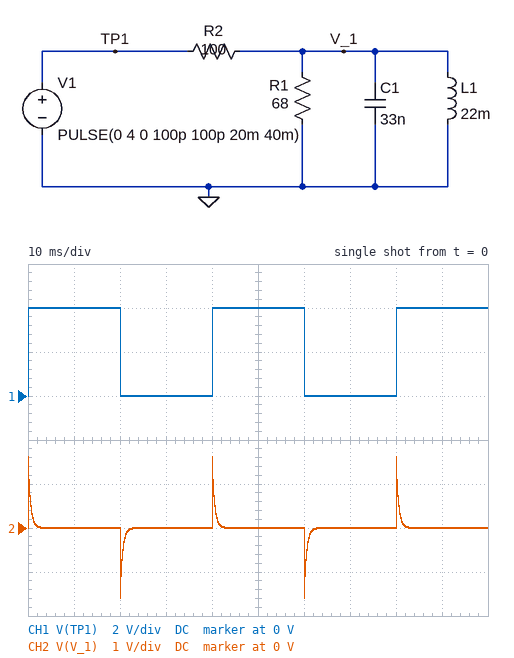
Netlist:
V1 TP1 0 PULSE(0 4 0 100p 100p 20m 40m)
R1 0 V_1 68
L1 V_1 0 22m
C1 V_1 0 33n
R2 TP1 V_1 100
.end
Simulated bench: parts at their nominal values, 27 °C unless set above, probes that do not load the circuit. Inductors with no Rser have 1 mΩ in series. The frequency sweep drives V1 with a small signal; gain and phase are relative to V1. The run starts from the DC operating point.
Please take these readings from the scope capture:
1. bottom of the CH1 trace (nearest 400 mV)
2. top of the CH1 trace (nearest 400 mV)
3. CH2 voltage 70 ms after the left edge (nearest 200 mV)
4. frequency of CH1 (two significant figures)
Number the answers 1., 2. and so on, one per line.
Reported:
1. 0 V
2. 4.0 V
3. 0 V
4. 25 Hz
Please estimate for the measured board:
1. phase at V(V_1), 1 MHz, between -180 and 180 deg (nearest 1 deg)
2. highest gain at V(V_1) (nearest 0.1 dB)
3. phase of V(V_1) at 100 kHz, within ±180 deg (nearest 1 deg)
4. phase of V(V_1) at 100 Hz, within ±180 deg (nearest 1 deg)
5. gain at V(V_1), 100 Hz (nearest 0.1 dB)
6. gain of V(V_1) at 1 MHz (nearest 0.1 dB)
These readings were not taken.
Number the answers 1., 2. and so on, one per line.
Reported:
1. -83 deg
2. -7.9 dB
3. -40 deg
4. 71 deg
5. -17.7 dB
6. -26.4 dB
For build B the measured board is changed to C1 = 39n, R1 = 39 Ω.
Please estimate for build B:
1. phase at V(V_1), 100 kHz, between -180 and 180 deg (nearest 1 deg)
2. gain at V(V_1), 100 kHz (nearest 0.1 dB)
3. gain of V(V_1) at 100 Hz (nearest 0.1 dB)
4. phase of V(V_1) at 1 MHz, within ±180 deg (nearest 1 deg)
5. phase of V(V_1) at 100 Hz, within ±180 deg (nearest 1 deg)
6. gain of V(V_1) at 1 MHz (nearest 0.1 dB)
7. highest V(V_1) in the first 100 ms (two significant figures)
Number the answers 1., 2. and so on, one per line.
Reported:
1. -34 deg
2. -12.7 dB
3. -18.1 dB
4. -82 deg
5. 64 deg
6. -27.9 dB
7. 1.1 V
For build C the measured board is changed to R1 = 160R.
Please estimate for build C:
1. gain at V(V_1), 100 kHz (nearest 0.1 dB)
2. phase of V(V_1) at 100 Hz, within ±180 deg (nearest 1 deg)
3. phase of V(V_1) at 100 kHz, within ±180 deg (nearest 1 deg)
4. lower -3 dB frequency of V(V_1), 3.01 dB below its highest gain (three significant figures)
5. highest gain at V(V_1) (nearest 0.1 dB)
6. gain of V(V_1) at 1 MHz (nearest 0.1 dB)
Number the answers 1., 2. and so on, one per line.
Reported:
1. -8.4 dB
2. 77 deg
3. -52 deg
4. 443 Hz
5. -4.2 dB
6. -26.4 dB
